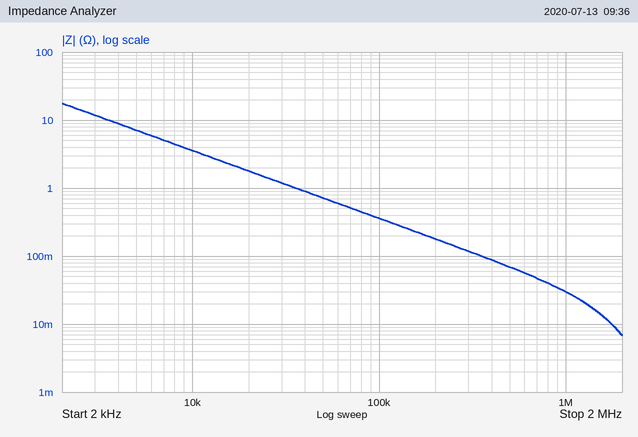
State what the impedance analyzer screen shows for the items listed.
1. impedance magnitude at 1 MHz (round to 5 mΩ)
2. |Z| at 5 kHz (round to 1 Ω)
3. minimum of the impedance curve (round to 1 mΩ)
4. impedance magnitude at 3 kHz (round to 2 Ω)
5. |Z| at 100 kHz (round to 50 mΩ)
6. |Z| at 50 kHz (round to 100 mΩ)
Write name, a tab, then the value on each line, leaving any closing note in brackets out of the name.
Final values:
impedance magnitude at 1 MHz	30 mΩ
|Z| at 5 kHz	7 Ω
minimum of the impedance curve	7 mΩ
impedance magnitude at 3 kHz	12 Ω
|Z| at 100 kHz	350 mΩ
|Z| at 50 kHz	700 mΩ
